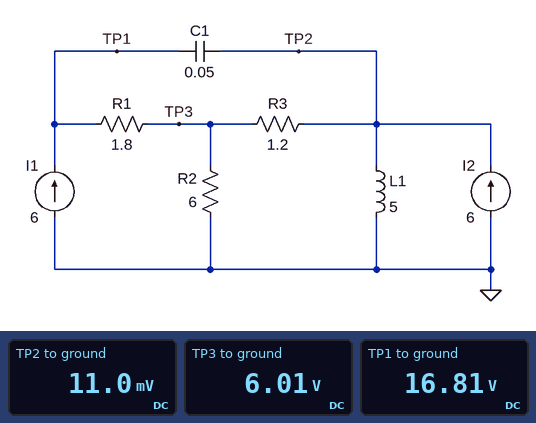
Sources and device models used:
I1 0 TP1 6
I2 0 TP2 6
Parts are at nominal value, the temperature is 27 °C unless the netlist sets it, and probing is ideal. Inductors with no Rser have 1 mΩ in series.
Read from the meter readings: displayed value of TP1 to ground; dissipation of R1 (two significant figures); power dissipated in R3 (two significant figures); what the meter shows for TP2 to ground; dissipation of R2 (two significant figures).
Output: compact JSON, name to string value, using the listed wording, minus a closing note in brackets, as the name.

{"displayed value of TP1 to ground": "16.81 V", "dissipation of R1": "65 W", "power dissipated in R3": "30 W", "what the meter shows for TP2 to ground": "11.0 mV", "dissipation of R2": "6.0 W"}
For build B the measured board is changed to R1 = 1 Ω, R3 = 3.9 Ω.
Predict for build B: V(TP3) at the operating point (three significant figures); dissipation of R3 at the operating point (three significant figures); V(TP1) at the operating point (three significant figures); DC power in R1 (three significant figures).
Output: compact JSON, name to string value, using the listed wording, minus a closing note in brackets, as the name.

{"V(TP3) at the operating point": "14.2 V", "dissipation of R3 at the operating point": "51.5 W", "V(TP1) at the operating point": "20.2 V", "DC power in R1": "36.0 W"}
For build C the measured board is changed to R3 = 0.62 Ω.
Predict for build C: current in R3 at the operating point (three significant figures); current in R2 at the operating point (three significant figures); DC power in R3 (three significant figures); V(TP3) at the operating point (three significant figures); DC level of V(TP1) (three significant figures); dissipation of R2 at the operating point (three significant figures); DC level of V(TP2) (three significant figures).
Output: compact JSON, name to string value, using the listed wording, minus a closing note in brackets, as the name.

{"current in R3 at the operating point": "5.44 A", "current in R2 at the operating point": "564 mA", "DC power in R3": "18.3 W", "V(TP3) at the operating point": "3.38 V", "DC level of V(TP1)": "14.2 V", "dissipation of R2 at the operating point": "1.91 W", "DC level of V(TP2)": "11.4 mV"}
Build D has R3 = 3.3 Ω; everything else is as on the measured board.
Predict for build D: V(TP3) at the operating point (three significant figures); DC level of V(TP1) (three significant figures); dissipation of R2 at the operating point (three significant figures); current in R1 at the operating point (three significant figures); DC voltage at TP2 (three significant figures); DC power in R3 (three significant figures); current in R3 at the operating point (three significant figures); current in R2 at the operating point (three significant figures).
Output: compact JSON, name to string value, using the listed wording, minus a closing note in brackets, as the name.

{"V(TP3) at the operating point": "12.8 V", "DC level of V(TP1)": "23.6 V", "dissipation of R2 at the operating point": "27.2 W", "current in R1 at the operating point": "6.00 A", "DC voltage at TP2": "9.87 mV", "DC power in R3": "49.4 W", "current in R3 at the operating point": "3.87 A", "current in R2 at the operating point": "2.13 A"}
